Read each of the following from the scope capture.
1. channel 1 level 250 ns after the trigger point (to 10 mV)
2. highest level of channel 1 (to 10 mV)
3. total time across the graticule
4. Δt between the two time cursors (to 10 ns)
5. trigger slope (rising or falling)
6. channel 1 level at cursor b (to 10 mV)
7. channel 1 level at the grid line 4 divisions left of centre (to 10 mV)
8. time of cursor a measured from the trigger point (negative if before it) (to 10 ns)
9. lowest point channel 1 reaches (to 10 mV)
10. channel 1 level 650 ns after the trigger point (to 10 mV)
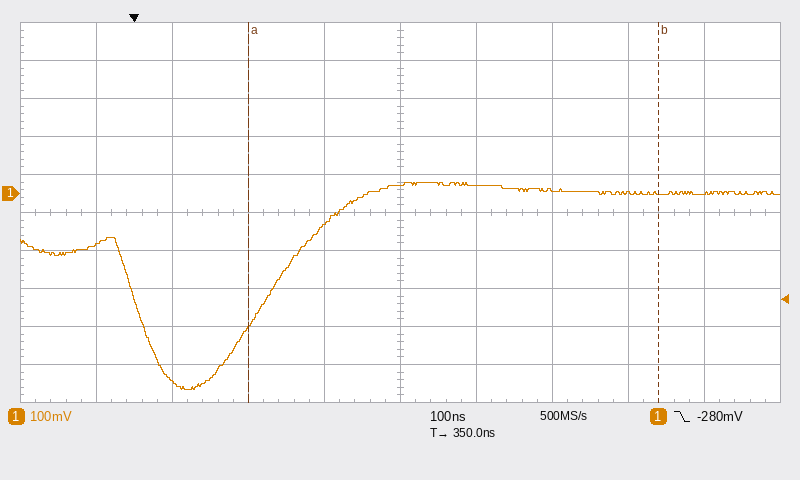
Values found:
-80 mV
30 mV
1 µs
540 ns
falling
0 mV
-130 mV
+150 ns
-520 mV
0 mV
